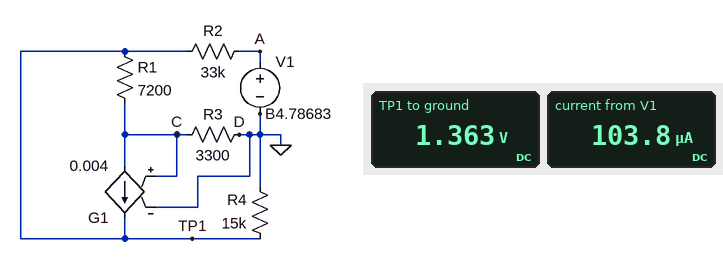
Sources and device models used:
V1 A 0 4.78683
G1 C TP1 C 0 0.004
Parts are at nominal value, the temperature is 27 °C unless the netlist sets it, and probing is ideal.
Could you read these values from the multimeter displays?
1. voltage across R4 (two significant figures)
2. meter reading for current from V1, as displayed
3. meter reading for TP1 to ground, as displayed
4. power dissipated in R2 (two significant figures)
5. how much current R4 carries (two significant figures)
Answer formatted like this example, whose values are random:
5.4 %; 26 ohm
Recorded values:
1.4 V; 103.8 µA; 1.363 V; 360 µW; 91 µA
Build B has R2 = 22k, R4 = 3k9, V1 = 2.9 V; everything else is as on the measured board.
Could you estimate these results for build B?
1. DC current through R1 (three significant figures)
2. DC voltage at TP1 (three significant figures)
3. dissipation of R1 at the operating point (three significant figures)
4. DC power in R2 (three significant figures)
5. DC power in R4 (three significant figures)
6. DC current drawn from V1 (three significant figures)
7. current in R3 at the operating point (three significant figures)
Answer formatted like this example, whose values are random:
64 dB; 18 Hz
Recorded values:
57.0 µA; 423 mV; 23.4 µW; 279 µW; 46.0 µW; 113 µA; 4.01 µA
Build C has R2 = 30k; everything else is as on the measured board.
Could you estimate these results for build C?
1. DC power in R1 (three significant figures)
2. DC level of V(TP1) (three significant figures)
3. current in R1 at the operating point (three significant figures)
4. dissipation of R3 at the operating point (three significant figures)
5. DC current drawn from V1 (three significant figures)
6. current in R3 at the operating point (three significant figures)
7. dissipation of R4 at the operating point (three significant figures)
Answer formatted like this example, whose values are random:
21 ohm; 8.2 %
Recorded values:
277 µW; 1.46 V; 196 µA; 629 nW; 111 µA; 13.8 µA; 142 µW
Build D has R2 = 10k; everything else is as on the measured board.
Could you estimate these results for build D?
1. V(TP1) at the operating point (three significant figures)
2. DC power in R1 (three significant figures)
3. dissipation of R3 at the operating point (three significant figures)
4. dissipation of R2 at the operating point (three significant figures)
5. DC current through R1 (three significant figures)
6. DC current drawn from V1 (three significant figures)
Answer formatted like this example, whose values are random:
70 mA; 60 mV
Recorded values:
2.72 V; 963 µW; 2.19 µW; 428 µW; 366 µA; 207 µA
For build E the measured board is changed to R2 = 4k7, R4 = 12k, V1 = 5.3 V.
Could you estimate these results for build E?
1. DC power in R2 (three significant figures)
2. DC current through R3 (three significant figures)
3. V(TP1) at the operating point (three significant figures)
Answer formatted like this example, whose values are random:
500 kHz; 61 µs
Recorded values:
551 µW; 35.0 µA; 3.69 V
